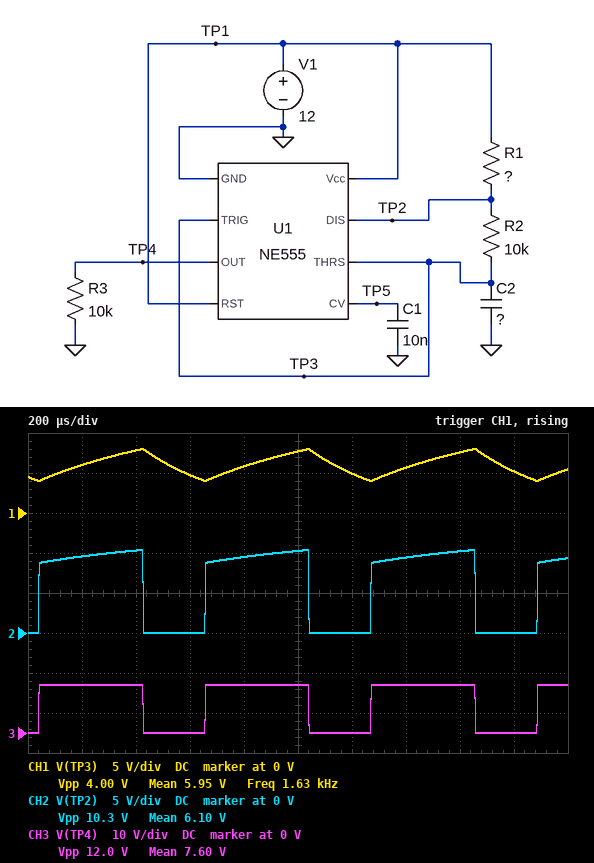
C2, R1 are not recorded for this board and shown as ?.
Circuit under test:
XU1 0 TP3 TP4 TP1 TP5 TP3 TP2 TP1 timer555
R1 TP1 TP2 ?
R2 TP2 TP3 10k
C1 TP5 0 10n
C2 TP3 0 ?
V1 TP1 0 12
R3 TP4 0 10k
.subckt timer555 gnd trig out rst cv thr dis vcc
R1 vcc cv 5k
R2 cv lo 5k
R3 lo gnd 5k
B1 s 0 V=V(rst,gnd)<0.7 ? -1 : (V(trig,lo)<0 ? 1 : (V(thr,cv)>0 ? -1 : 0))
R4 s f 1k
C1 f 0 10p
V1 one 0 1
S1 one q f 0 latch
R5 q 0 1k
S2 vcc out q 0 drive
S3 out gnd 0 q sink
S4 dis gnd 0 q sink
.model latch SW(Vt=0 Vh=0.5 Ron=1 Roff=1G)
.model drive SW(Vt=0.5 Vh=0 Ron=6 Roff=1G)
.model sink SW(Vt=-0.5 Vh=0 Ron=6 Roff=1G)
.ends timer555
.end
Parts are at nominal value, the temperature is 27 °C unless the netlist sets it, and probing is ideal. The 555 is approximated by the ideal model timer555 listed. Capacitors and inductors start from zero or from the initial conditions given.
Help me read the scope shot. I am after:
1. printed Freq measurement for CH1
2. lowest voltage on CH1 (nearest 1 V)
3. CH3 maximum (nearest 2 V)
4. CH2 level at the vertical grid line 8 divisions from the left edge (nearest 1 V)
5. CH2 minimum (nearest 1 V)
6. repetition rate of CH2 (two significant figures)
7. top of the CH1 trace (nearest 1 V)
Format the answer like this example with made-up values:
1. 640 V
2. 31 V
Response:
1. 1.63 kHz
2. 4 V
3. 12 V
4. 10 V
5. 0 V
6. 1.6 kHz
7. 8 V
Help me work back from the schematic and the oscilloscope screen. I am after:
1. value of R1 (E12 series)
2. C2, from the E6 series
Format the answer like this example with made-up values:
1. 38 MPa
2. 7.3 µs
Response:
1. 6.8 kΩ
2. 33 nF
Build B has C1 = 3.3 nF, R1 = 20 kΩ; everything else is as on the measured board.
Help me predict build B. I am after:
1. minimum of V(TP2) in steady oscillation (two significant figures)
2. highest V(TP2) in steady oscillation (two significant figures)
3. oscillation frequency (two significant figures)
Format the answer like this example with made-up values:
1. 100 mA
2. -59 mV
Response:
1. 6.0 mV
2. 9.3 V
3. 1.1 kHz
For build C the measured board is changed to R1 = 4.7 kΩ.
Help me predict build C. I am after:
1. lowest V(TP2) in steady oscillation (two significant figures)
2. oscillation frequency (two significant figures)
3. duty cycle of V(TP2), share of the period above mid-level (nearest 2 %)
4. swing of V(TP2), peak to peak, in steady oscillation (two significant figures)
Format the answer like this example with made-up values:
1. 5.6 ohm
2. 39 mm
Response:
1. 18 mV
2. 1.8 kHz
3. 60 %
4. 11 V
